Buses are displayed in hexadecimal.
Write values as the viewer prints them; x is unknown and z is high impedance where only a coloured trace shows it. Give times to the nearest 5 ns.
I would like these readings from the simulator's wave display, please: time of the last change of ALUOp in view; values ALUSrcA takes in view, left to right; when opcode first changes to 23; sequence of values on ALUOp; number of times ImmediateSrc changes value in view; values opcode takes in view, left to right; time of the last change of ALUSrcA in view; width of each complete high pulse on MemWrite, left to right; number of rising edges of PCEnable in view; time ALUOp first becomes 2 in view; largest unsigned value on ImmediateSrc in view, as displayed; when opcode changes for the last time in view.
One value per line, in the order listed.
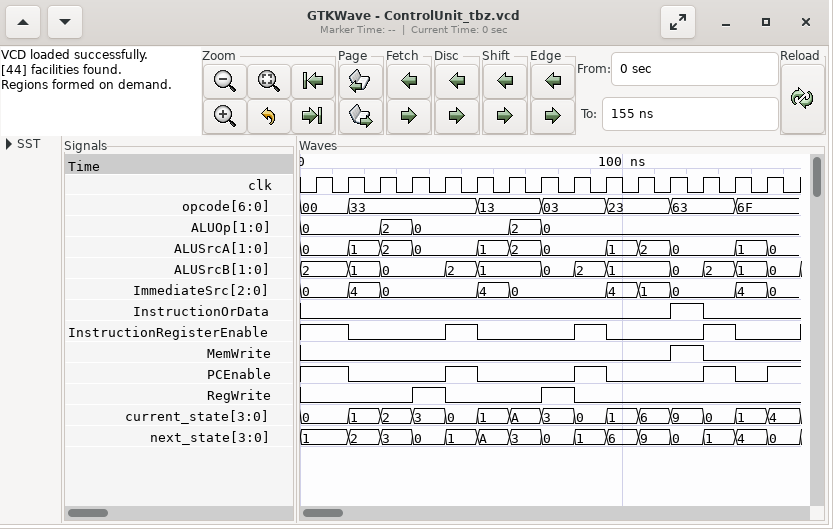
75 ns
0, 1, 2, 0, 1, 2, 0, 1, 2, 0, 1, 0
95 ns
0, 2, 0, 2, 0
9
00, 33, 13, 03, 23, 63, 6F
145 ns
10 ns
4
25 ns
4
135 ns
